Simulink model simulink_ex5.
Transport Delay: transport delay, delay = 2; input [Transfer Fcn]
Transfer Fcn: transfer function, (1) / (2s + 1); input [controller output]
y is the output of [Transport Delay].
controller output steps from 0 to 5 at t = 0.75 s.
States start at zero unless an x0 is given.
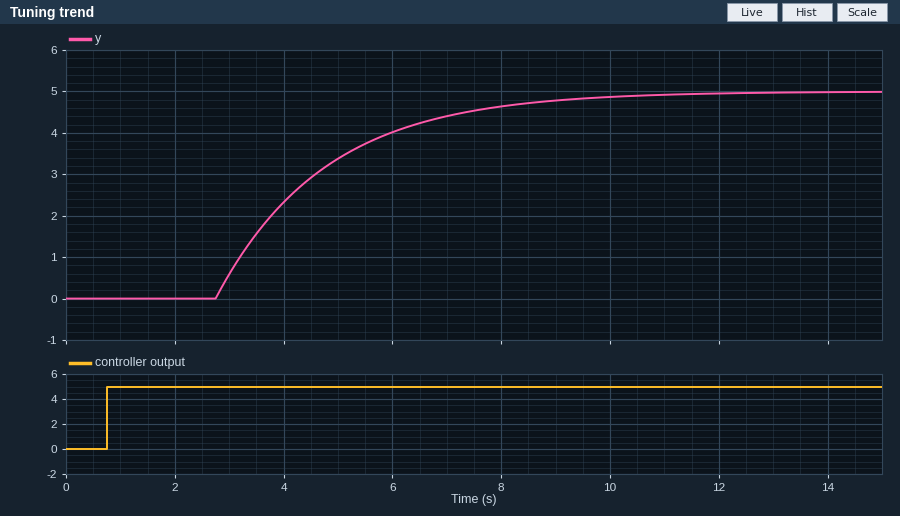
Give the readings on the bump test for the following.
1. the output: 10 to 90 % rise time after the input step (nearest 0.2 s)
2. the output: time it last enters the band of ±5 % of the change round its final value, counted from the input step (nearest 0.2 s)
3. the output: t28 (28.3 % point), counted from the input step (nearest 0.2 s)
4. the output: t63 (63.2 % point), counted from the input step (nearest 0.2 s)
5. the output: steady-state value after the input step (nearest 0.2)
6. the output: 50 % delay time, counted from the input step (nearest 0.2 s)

4.4 s
8.0 s
2.6 s
4.0 s
5.0
3.4 s
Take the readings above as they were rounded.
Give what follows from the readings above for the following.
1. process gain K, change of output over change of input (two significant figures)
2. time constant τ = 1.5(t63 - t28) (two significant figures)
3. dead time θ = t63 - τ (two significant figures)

1.0
2.1 s
1.9 s
